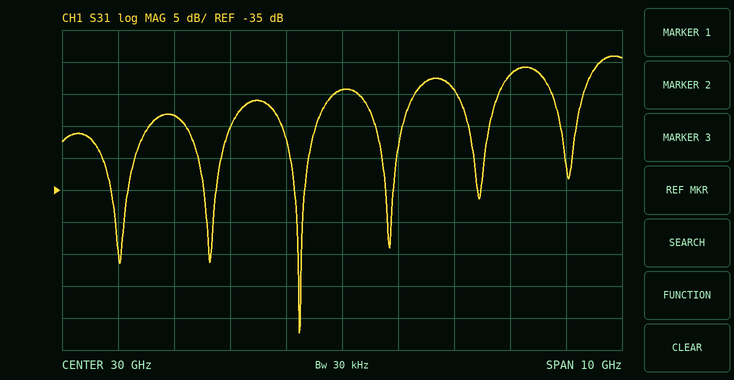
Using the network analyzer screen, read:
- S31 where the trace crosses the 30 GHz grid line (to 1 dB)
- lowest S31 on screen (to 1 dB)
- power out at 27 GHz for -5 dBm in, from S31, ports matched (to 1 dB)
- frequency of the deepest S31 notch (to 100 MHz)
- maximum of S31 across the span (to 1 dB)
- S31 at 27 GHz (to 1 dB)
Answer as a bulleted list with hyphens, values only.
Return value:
- -19 dB
- -57 dB
- -28 dBm
- 29.2 GHz
- -14 dB
- -23 dB
